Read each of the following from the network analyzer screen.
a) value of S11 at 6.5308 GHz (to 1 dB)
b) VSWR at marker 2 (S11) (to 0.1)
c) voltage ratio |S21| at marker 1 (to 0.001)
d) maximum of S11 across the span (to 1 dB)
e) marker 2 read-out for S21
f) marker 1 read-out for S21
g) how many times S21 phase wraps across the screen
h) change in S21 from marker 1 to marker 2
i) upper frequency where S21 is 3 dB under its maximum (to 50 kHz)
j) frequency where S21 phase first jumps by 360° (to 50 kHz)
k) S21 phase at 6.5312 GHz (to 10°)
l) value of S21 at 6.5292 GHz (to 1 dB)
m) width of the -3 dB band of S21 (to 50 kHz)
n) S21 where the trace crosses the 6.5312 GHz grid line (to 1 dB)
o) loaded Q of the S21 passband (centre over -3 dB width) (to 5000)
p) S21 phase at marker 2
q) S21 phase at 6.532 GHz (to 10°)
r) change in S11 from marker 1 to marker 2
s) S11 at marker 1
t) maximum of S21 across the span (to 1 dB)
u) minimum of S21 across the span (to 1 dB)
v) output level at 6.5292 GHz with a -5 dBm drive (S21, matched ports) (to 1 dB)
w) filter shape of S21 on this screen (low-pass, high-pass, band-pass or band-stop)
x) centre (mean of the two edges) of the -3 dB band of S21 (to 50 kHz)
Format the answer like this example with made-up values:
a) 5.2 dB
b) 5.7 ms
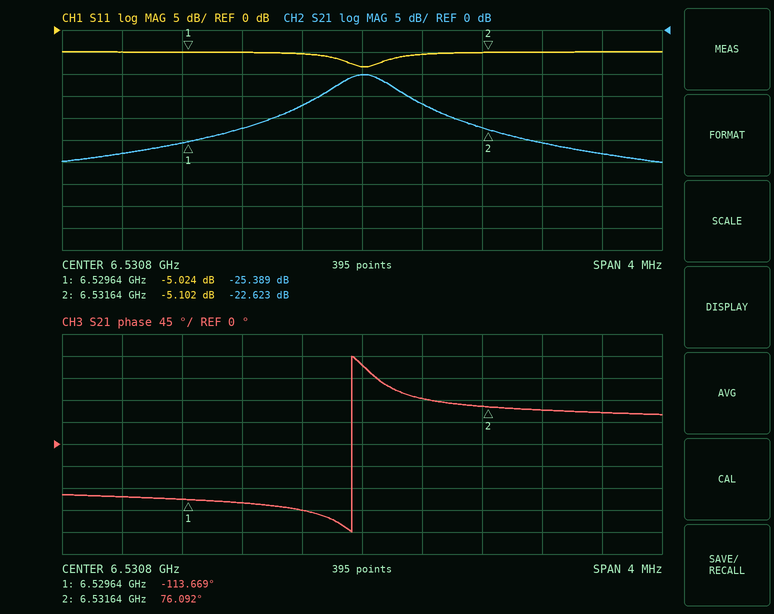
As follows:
a) -8 dB
b) 3.5
c) 0.054
d) -5 dB
e) -22.623 dB
f) -25.389 dB
g) 1
h) 2.766 dB
i) 6.53100 GHz
j) 6.53075 GHz
k) 90°
l) -28 dB
m) 400 kHz
n) -17 dB
o) 15000
p) 76.092°
q) 70°
r) -0.078 dB
s) -5.024 dB
t) -10 dB
u) -30 dB
v) -33 dBm
w) band-pass
x) 6.53080 GHz
